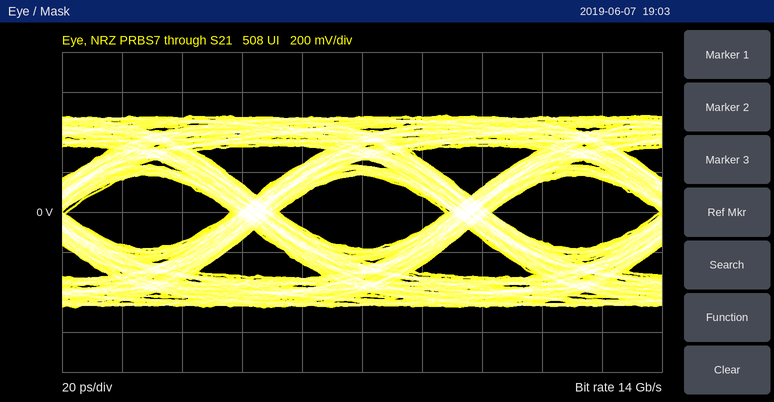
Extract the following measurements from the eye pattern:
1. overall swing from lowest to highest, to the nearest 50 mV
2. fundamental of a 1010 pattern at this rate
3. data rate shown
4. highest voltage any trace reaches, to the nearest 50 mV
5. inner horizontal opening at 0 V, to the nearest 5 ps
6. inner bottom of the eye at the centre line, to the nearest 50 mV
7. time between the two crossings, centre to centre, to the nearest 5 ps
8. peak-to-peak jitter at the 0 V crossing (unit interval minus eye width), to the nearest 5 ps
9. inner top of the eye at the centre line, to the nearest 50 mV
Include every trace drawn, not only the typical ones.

950 mV
7 GHz
14 Gb/s
500 mV
55 ps
-200 mV
70 ps
15 ps
200 mV
